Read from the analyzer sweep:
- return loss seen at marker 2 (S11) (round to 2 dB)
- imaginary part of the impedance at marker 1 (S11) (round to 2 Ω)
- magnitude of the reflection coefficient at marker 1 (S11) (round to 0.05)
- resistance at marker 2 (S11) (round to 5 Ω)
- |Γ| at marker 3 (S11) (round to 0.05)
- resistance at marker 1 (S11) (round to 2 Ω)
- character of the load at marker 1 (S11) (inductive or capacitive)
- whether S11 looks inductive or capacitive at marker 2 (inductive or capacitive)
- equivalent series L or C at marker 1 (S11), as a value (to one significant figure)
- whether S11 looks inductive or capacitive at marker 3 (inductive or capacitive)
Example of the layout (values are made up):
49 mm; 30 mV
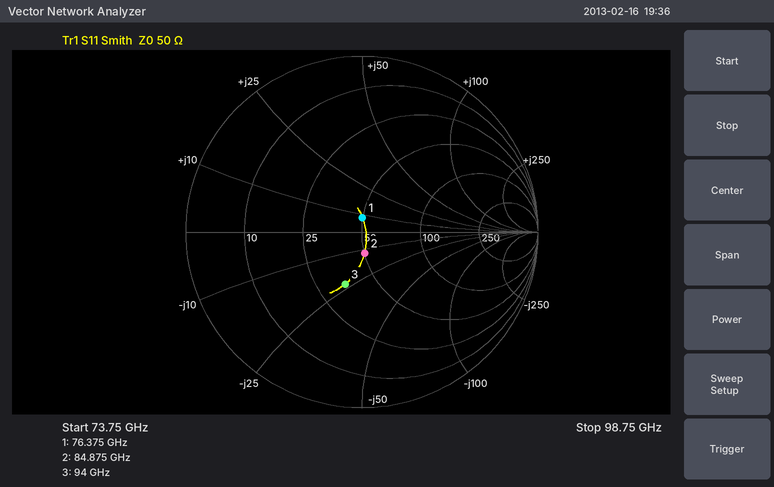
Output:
18 dB; +8 Ω; 0.10; 50 Ω; 0.30; 50 Ω; inductive; capacitive; 20 pH; capacitive
